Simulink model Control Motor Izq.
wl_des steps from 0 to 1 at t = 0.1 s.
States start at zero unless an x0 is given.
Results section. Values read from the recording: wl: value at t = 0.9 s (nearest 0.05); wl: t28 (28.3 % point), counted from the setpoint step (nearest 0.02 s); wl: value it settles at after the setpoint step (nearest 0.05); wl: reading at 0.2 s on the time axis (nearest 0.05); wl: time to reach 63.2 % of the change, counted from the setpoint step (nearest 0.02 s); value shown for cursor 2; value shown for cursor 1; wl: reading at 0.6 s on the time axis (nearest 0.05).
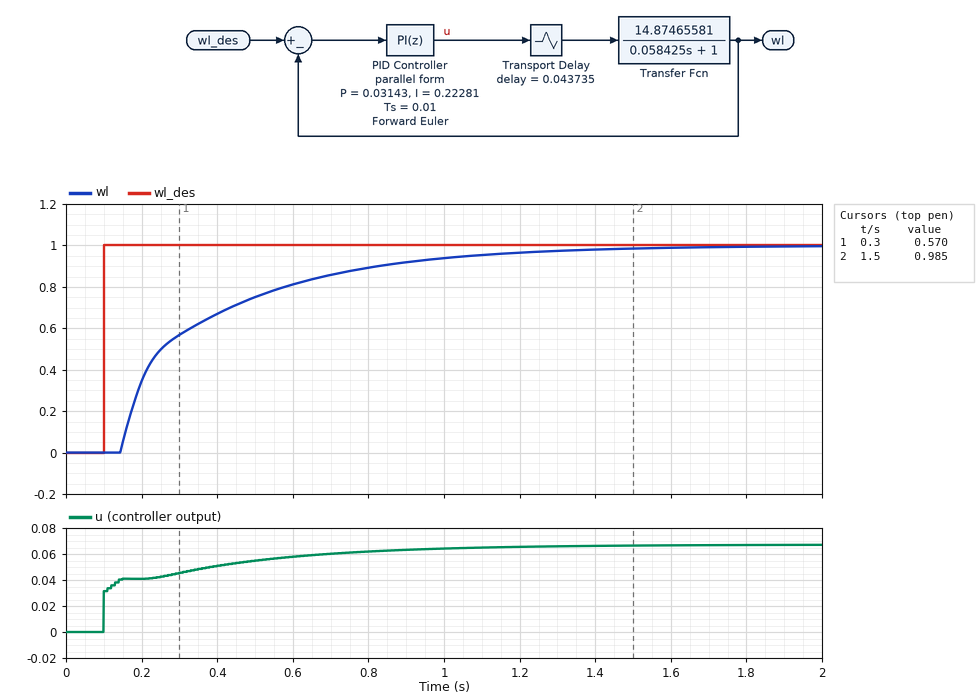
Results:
0.90
0.08 s
1.00
0.35
0.26 s
0.985
0.570
0.80
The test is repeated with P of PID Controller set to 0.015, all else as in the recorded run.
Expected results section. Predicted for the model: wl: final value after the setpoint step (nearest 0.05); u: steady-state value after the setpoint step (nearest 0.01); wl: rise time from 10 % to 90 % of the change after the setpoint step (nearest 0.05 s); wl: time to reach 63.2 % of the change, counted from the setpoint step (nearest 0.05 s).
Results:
1.00
0.07
0.55 s
0.30 s
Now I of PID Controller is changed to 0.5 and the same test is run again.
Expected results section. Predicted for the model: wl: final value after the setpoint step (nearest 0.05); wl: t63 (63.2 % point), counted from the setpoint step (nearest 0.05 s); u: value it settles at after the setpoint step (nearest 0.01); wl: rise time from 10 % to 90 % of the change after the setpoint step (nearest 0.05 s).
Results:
1.00
0.15 s
0.07
0.15 s
